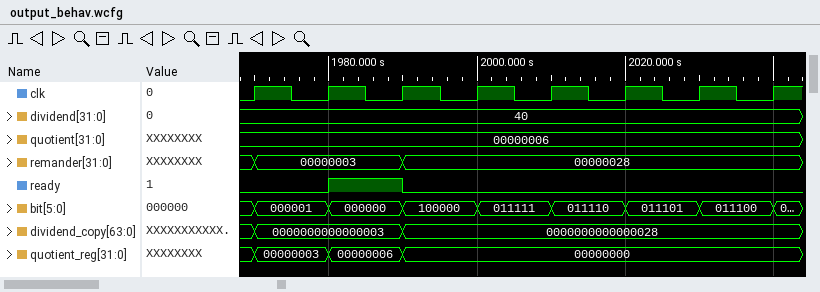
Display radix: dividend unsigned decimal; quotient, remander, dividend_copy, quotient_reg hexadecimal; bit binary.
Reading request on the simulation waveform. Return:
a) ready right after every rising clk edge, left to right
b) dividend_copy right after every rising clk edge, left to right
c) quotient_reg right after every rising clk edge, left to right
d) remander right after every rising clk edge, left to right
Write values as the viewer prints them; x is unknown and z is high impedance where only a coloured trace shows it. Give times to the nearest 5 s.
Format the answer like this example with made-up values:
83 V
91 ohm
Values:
0 1 0 0 0 0 0 0
0000000000000003, 0000000000000003, 0000000000000028, 0000000000000028, 0000000000000028, 0000000000000028, 0000000000000028, 0000000000000028
00000003, 00000006, 00000000, 00000000, 00000000, 00000000, 00000000, 00000000
00000003, 00000003, 00000028, 00000028, 00000028, 00000028, 00000028, 00000028
